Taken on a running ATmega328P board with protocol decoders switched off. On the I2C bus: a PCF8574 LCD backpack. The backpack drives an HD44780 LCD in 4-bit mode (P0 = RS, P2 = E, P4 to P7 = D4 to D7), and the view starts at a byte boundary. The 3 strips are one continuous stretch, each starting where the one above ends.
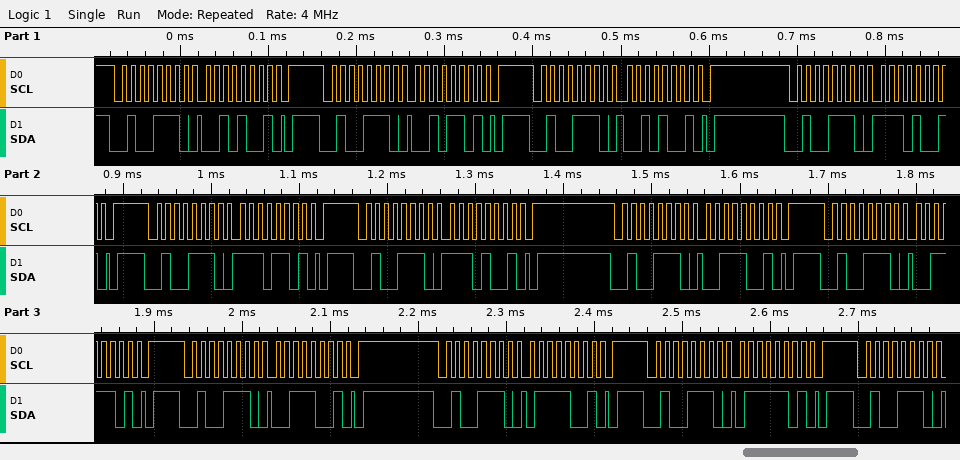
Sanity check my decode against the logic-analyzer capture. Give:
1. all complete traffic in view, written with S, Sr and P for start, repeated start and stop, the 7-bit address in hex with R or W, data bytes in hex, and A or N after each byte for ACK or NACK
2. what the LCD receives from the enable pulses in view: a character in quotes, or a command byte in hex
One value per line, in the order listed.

S 27W A 29 A P S 27W A 2D A P S 27W A 29 A P S 27W A E9 A P S 27W A ED A P S 27W A E9 A P S 27W A 39 A P S 27W A 3D A P S 27W A 39 A P S 27W A 79 A P S 27W A 7D A P S 27W A
'.'
